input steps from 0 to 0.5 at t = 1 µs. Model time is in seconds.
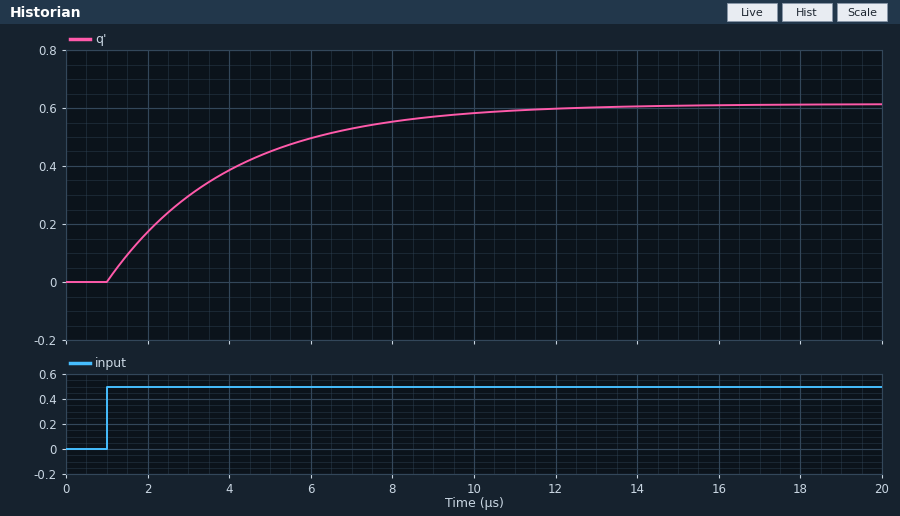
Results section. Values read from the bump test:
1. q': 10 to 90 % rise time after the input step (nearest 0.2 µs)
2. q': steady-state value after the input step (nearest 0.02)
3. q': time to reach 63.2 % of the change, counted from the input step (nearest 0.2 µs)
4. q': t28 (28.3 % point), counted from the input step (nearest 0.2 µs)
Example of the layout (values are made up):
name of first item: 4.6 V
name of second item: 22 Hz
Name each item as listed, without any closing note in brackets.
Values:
q': 10 to 90 % rise time after the input step: 6.6 µs
q': steady-state value after the input step: 0.62
q': time to reach 63.2 % of the change, counted from the input step: 3.0 µs
q': t28 (28.3 % point), counted from the input step: 1.0 µs
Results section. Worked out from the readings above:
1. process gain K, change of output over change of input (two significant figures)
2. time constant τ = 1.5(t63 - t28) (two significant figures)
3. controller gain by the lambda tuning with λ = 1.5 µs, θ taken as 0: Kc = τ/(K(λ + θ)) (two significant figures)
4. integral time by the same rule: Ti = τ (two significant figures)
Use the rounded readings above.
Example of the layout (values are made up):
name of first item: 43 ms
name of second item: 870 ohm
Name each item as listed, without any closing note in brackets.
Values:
process gain K, change of output over change of input: 1.2
time constant τ = 1.5(t63 - t28): 3.0 µs
controller gain by the lambda tuning with λ = 1.5 µs, θ taken as 0: Kc = τ/(K(λ + θ)): 1.7
integral time by the same rule: Ti = τ: 3.0 µs
